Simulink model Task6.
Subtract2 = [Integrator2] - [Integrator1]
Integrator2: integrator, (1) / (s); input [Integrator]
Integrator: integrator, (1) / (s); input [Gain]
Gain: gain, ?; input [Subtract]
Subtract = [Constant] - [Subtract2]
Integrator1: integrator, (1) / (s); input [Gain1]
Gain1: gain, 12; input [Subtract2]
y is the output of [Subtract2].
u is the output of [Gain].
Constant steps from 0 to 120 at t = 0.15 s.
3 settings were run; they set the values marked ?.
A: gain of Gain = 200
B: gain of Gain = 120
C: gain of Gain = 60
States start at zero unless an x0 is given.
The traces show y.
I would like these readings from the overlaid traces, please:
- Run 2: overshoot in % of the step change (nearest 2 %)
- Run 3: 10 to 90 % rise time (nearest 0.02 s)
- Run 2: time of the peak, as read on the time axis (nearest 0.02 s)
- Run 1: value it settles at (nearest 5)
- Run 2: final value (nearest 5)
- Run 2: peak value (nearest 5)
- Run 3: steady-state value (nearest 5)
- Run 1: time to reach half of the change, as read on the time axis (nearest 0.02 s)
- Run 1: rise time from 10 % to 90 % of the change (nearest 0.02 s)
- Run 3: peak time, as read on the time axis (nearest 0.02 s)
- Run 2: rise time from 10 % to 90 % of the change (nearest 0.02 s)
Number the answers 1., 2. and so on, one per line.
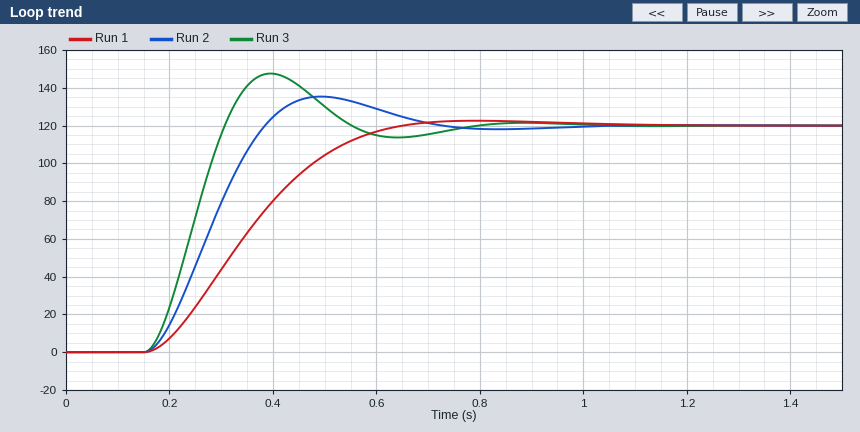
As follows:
1. 12 %
2. 0.10 s
3. 0.50 s
4. 120
5. 120
6. 135
7. 120
8. 0.34 s
9. 0.30 s
10. 0.40 s
11. 0.16 s
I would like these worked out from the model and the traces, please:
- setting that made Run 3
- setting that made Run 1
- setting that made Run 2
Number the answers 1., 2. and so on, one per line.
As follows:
1. A
2. C
3. B
